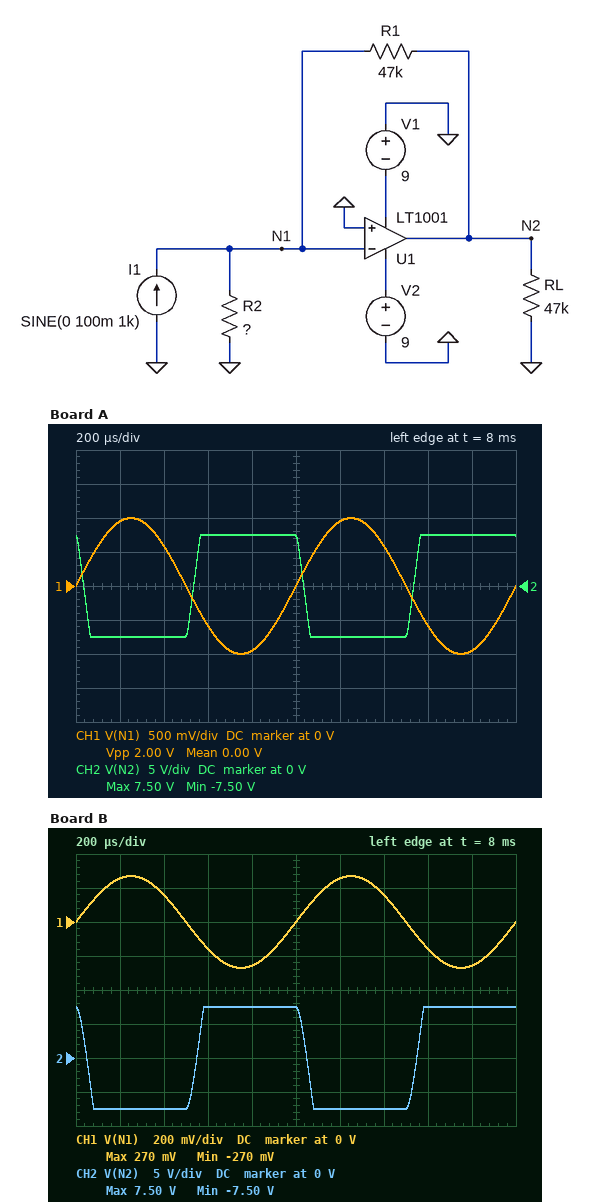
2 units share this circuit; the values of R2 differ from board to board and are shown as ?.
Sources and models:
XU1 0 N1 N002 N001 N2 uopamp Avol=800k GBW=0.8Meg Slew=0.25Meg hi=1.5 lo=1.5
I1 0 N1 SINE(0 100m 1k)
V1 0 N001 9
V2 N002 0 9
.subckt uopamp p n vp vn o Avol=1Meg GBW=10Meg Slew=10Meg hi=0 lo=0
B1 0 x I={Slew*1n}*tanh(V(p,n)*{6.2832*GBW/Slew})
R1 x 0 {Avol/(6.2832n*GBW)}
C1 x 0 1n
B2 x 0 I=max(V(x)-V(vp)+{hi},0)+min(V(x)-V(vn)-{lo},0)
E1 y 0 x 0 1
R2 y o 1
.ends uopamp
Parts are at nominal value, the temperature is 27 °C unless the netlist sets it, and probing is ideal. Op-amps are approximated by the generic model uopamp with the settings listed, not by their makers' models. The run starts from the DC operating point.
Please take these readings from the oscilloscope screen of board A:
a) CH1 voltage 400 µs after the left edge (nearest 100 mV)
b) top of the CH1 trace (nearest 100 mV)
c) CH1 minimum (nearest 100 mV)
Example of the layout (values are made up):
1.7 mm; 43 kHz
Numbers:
600 mV; 1.0 V; -1.0 V
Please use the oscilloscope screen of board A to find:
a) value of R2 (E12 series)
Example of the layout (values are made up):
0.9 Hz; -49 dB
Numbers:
10 Ω
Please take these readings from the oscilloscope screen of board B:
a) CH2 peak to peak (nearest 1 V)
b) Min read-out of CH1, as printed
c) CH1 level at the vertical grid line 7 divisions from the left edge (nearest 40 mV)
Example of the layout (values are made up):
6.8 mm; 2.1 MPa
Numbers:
15 V; -270 mV; 160 mV
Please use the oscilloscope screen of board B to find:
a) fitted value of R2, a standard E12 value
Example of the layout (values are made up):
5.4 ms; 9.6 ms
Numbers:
2.7 Ω
